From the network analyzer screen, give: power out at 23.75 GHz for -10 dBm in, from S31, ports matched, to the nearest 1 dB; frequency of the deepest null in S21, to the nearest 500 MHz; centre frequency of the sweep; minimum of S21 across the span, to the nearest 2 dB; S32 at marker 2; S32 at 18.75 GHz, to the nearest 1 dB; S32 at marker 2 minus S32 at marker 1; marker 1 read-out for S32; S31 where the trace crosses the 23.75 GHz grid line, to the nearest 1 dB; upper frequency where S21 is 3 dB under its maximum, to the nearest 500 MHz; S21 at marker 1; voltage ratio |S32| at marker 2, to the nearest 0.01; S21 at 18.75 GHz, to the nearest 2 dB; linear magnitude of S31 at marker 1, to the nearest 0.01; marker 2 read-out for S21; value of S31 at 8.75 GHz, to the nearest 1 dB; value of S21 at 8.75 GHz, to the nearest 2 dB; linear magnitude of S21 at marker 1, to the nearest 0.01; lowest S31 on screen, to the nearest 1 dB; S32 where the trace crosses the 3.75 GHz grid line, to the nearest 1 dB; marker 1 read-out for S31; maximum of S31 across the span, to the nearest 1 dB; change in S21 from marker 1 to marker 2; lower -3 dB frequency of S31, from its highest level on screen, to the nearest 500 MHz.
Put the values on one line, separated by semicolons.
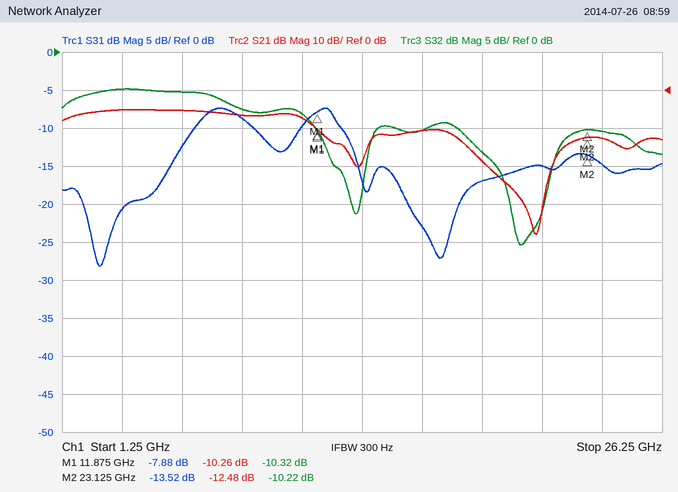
-25 dBm; 21.0 GHz; 13.75 GHz; -38 dB; -10.22 dB; -13 dB; 0.10 dB; -10.32 dB; -15 dB; 11.5 GHz; -10.26 dB; 0.31; -18 dB; 0.40; -12.48 dB; -9 dB; -6 dB; 0.31; -28 dB; -5 dB; -7.88 dB; -7 dB; -2.22 dB; 6.5 GHz
